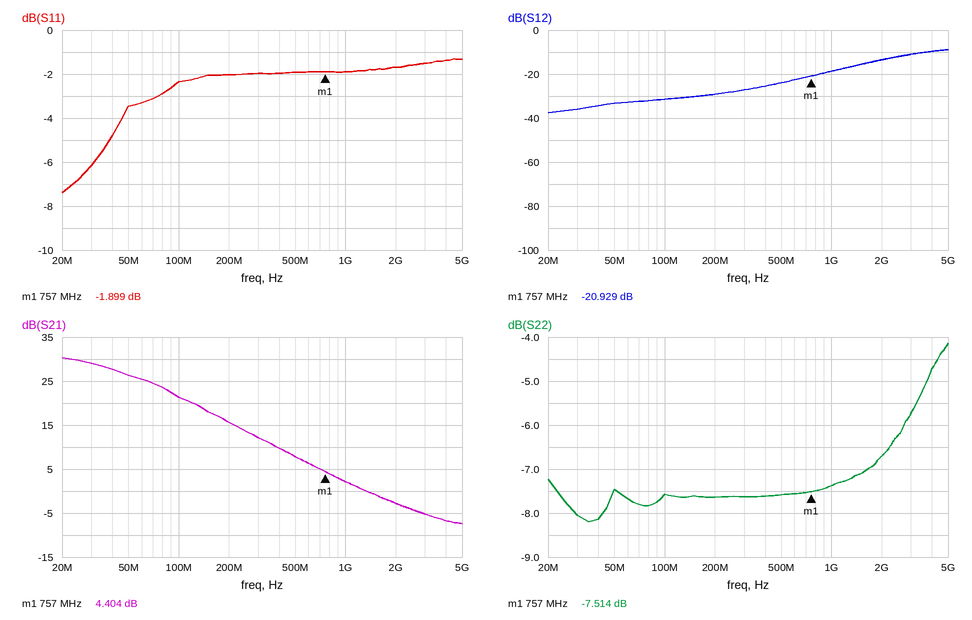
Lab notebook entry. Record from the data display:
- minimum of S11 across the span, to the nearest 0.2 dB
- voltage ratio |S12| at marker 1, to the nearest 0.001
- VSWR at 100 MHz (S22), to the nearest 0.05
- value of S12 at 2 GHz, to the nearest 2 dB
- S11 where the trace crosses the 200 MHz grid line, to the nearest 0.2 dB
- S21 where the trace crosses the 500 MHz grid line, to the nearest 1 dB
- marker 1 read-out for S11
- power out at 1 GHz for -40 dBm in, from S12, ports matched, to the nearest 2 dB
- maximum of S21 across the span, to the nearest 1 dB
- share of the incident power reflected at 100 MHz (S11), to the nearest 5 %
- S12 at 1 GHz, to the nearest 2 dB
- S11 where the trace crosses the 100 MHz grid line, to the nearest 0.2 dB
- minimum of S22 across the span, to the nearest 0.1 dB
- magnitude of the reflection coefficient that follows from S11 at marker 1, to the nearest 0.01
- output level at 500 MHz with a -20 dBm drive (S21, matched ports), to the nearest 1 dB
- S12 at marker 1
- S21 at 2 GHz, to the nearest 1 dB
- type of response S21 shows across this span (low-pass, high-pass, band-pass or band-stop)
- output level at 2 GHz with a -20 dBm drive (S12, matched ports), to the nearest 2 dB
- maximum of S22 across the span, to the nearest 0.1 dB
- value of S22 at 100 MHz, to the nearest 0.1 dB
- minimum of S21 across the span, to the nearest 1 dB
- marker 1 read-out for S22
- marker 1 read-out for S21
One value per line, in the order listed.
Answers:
-7.4 dB
0.090
2.45
-14 dB
-2.0 dB
8 dB
-1.899 dB
-58 dBm
30 dB
60 %
-18 dB
-2.4 dB
-8.2 dB
0.80
-12 dBm
-20.929 dB
-3 dB
low-pass
-34 dBm
-4.1 dB
-7.6 dB
-7 dB
-7.514 dB
4.404 dB
